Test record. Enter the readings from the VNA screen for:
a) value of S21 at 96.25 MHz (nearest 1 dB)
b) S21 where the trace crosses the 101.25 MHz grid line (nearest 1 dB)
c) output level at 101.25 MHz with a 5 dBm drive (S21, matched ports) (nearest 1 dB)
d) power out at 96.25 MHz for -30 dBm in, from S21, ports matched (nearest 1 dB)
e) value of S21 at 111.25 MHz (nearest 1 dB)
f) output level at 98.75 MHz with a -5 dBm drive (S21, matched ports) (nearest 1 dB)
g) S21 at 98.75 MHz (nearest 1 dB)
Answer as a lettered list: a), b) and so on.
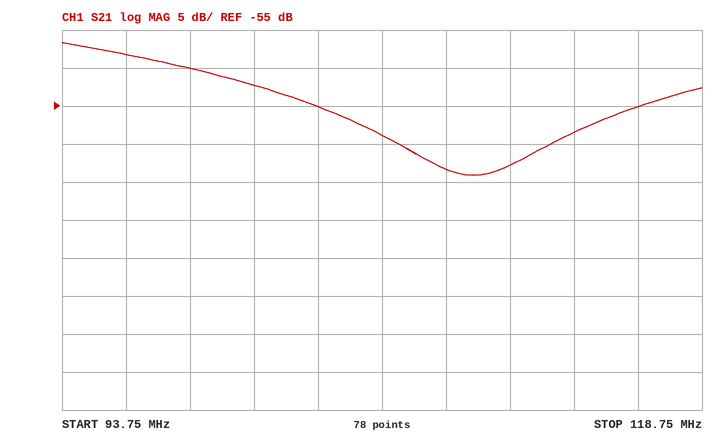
a) -48 dB
b) -52 dB
c) -47 dBm
d) -78 dBm
e) -63 dB
f) -55 dBm
g) -50 dB
